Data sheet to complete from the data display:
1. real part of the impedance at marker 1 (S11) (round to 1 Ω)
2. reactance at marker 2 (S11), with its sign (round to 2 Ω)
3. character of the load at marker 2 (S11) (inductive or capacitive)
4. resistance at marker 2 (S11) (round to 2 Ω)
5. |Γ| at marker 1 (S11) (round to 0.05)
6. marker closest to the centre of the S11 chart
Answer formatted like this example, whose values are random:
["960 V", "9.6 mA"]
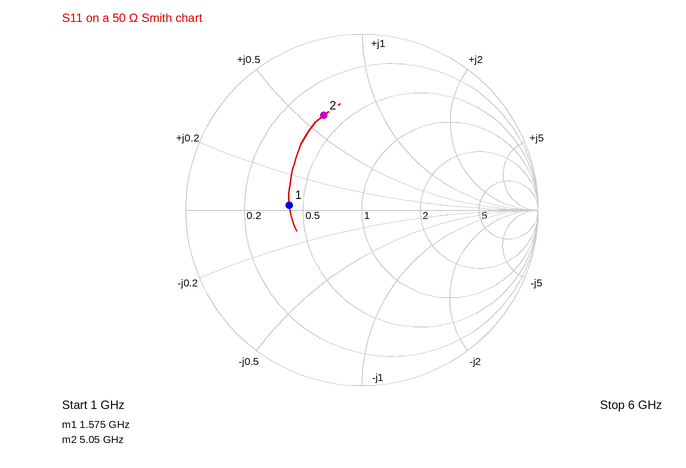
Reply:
["21 Ω", "+30 Ω", "inductive", "18 Ω", "0.40", "marker 1"]
